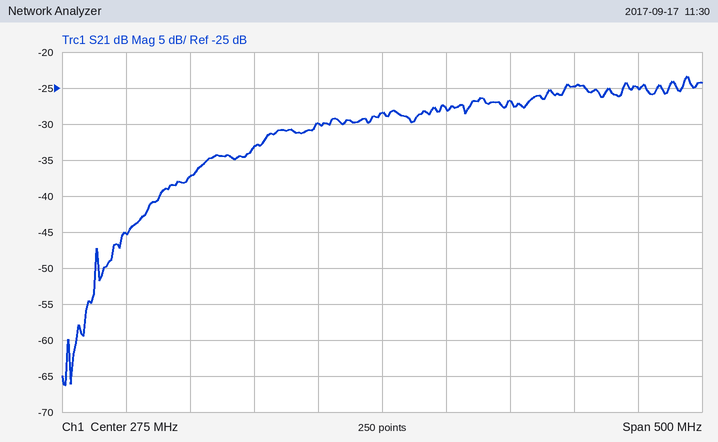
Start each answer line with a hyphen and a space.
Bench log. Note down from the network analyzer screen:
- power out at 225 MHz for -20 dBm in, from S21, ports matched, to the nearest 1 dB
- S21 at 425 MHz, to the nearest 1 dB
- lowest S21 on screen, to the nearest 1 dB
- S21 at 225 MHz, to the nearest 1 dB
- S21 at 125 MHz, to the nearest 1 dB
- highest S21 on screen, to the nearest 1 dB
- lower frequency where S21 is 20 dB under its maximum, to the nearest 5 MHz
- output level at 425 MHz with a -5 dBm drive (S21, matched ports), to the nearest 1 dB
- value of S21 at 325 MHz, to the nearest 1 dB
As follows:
- -50 dBm
- -25 dB
- -66 dB
- -30 dB
- -37 dB
- -23 dB
- 85 MHz
- -30 dBm
- -28 dB
